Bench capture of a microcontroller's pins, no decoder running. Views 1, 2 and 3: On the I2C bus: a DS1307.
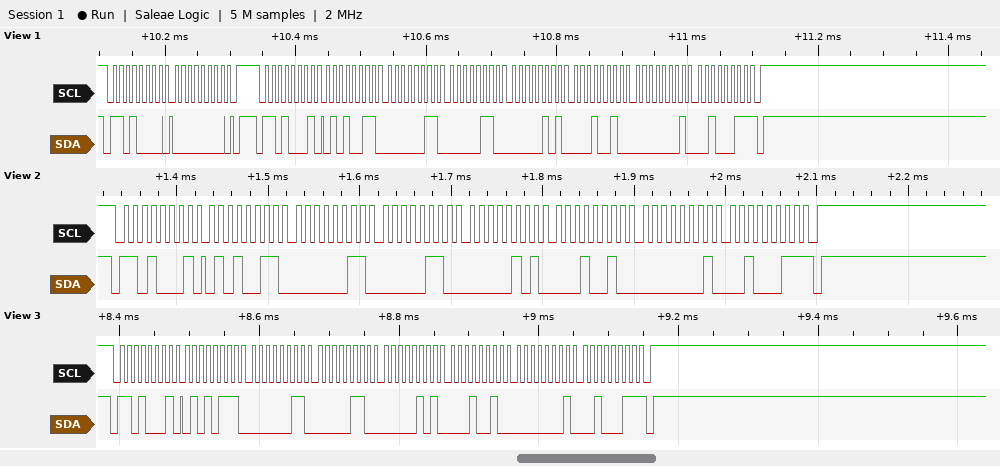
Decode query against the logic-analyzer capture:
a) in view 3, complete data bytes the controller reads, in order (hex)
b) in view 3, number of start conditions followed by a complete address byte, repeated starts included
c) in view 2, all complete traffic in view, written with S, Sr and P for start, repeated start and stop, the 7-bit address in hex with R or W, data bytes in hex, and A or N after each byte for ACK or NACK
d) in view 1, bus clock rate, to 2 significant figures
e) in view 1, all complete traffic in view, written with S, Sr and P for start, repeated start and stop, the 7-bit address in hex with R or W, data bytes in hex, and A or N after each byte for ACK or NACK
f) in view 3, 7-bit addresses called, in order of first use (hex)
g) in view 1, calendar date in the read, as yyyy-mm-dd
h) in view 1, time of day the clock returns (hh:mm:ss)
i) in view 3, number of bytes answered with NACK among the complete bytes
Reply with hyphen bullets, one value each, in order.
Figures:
- 57 03 06 05 12 01 23
- 1
- S 68R A 53 A 03 A 06 A 05 A 12 A 01 A 23 N P
- 100 kHz
- S 68W A 00 A P S 68R A 53 A 03 A 06 A 05 A 12 A 01 A 23 N P
- 0x68
- 2023-01-12
- 06:03:53
- 1
